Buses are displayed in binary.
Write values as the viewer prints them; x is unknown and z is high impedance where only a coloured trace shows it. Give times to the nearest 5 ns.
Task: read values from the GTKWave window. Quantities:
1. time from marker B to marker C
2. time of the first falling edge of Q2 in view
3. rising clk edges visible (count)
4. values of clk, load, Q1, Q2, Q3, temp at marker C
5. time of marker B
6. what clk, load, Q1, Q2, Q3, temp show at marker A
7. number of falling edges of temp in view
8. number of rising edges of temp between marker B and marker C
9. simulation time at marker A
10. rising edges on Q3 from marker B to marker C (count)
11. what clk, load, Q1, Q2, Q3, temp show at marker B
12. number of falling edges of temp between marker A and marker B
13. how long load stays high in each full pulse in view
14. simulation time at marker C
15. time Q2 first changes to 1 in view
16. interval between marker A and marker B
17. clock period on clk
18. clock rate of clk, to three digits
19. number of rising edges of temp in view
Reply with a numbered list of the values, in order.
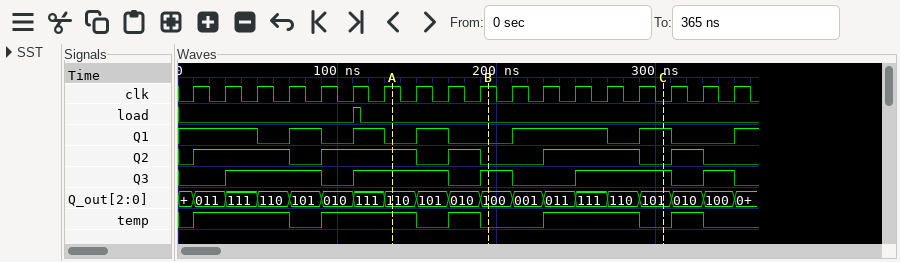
1. 110 ns
2. 70 ns
3. 18
4. clk=0, load=0, Q1=1, Q2=0, Q3=1, temp=0
5. 195 ns
6. clk=1, load=0, Q1=0, Q2=1, Q3=1, temp=1
7. 5
8. 1
9. 135 ns
10. 1
11. clk=1, load=0, Q1=0, Q2=0, Q3=1, temp=0
12. 2
13. 5 ns
14. 305 ns
15. 10 ns
16. 60 ns
17. 20 ns
18. 50.0 MHz
19. 5
